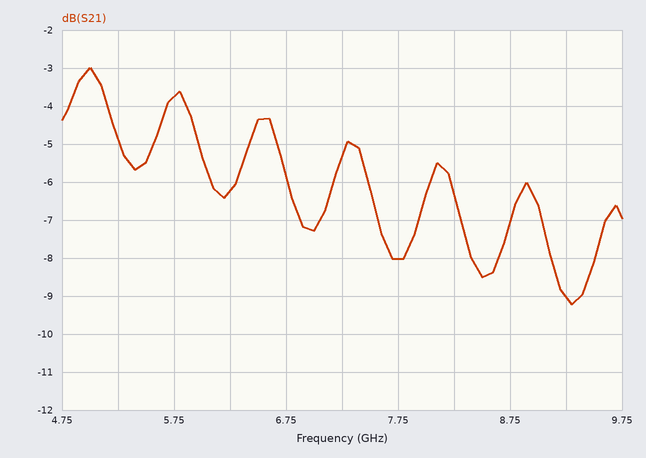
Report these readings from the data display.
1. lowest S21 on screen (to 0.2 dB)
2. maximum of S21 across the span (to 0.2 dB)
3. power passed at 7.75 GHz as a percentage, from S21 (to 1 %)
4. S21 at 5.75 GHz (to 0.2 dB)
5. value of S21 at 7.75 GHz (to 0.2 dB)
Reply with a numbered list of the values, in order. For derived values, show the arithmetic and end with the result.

1. -9.2 dB
2. -3.0 dB
3. 10^(-8/10) ≈ 16 %
4. -3.8 dB
5. -8.0 dB
